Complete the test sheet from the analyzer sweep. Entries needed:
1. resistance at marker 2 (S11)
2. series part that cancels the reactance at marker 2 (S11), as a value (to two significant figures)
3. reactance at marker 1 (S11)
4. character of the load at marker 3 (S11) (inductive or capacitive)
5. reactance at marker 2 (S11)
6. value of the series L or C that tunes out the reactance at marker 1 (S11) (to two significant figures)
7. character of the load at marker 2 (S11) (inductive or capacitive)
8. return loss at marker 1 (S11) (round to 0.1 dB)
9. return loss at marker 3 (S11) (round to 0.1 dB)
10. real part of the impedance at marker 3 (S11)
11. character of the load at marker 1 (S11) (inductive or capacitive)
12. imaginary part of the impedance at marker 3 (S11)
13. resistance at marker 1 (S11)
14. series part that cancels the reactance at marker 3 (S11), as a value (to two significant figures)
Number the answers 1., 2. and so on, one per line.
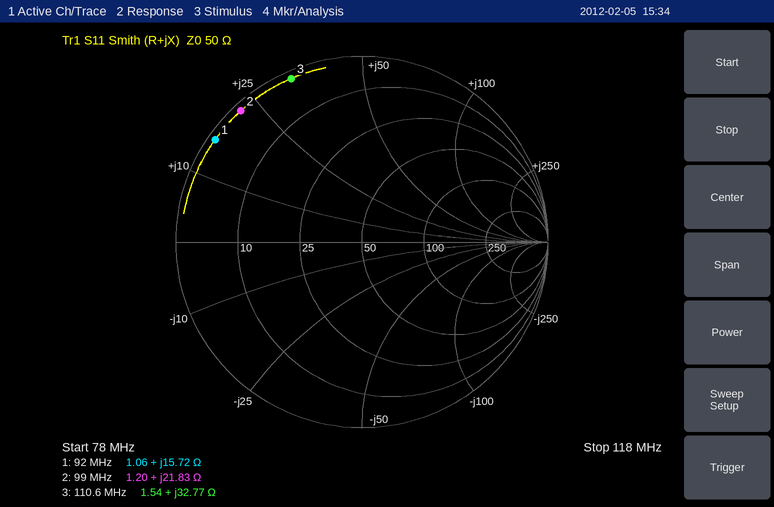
1. 1.20 Ω
2. 74 pF
3. +15.72 Ω
4. inductive
5. +21.83 Ω
6. 110 pF
7. inductive
8. 0.3 dB
9. 0.4 dB
10. 1.54 Ω
11. inductive
12. +32.77 Ω
13. 1.06 Ω
14. 44 pF
